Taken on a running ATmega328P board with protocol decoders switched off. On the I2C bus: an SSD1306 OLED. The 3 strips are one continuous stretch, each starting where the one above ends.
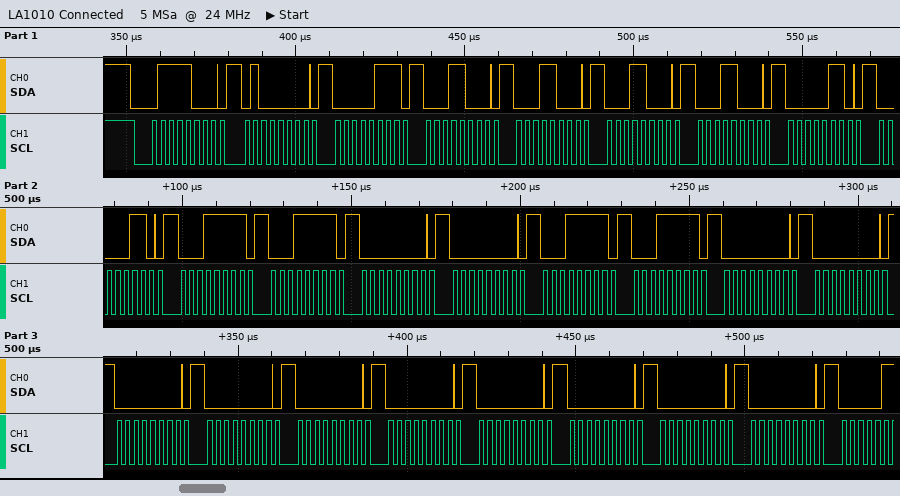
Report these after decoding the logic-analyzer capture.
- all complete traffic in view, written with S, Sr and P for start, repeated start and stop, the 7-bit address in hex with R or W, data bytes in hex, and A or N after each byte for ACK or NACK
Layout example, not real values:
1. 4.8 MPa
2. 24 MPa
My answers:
1. S 3CW A 40 A 07 A 18 A 18 A 18 A 18 A 06 A 06 A 1F A 1F A 00 A 00 A 1F A 1F A 00 A 00 A 00 A 00 A 00 A 00 A 00 A 00 A 00 A 00 A
